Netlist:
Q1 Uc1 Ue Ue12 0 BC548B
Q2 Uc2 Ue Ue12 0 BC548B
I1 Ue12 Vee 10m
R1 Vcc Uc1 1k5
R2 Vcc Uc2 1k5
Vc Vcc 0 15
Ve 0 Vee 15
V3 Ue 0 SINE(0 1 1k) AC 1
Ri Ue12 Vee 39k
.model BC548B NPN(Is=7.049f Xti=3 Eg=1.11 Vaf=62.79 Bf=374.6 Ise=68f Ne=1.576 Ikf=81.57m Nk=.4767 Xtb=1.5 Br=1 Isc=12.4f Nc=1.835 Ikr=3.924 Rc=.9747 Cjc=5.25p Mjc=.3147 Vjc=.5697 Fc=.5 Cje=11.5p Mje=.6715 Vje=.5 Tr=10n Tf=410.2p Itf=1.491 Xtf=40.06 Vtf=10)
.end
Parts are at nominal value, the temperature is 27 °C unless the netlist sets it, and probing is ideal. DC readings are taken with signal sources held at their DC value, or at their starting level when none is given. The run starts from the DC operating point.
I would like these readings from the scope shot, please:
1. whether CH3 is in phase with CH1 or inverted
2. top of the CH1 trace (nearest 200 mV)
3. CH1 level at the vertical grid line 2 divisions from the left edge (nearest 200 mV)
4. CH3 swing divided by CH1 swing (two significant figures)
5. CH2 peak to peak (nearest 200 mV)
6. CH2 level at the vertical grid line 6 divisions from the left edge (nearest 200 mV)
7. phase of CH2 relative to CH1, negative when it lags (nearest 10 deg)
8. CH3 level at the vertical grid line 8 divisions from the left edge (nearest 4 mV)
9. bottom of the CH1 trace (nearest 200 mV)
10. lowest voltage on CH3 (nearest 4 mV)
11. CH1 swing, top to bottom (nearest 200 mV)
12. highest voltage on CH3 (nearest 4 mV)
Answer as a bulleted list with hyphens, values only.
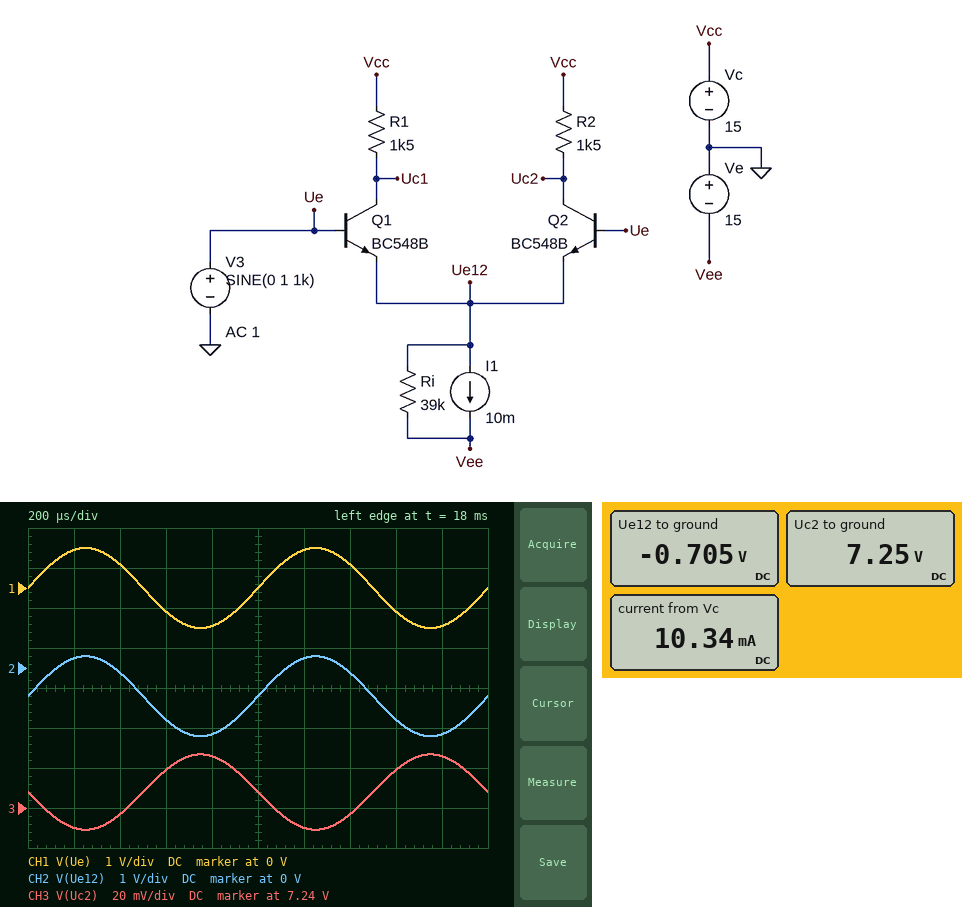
- inverted
- 1.0 V
- 600 mV
- 0.019
- 2.0 V
- 200 mV
- 0 deg
- 7.260 V
- -1.0 V
- 7.228 V
- 2.0 V
- 7.268 V
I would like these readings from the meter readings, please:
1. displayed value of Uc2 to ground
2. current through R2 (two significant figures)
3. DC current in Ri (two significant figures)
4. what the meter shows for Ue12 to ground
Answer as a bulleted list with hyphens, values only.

- 7.25 V
- 5.2 mA
- 370 µA
- -0.705 V
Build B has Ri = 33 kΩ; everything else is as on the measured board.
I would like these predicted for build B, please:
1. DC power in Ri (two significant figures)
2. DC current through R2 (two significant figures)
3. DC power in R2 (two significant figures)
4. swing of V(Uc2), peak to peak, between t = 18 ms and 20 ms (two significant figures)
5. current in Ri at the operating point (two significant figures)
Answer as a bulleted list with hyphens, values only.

- 6.2 mW
- 5.2 mA
- 41 mW
- 45 mV
- 430 µA
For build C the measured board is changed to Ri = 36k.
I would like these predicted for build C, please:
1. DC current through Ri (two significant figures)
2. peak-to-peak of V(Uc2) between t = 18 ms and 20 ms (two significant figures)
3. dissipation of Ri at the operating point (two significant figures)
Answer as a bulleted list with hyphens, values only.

- 400 µA
- 41 mV
- 5.7 mW
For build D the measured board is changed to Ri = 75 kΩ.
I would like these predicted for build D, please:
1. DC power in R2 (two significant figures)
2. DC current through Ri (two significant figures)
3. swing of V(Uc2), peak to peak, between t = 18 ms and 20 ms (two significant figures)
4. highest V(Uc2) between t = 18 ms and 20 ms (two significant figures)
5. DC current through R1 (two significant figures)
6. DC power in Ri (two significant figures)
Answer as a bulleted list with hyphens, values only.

- 39 mW
- 190 µA
- 19 mV
- 7.4 V
- 5.1 mA
- 2.7 mW
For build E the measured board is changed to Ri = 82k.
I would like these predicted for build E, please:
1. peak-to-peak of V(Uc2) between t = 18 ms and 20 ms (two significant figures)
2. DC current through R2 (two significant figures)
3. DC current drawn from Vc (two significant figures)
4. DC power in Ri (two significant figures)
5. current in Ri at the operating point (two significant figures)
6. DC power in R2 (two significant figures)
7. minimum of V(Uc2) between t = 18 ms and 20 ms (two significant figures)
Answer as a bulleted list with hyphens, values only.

- 18 mV
- 5.1 mA
- 10 mA
- 2.5 mW
- 170 µA
- 39 mW
- 7.4 V
